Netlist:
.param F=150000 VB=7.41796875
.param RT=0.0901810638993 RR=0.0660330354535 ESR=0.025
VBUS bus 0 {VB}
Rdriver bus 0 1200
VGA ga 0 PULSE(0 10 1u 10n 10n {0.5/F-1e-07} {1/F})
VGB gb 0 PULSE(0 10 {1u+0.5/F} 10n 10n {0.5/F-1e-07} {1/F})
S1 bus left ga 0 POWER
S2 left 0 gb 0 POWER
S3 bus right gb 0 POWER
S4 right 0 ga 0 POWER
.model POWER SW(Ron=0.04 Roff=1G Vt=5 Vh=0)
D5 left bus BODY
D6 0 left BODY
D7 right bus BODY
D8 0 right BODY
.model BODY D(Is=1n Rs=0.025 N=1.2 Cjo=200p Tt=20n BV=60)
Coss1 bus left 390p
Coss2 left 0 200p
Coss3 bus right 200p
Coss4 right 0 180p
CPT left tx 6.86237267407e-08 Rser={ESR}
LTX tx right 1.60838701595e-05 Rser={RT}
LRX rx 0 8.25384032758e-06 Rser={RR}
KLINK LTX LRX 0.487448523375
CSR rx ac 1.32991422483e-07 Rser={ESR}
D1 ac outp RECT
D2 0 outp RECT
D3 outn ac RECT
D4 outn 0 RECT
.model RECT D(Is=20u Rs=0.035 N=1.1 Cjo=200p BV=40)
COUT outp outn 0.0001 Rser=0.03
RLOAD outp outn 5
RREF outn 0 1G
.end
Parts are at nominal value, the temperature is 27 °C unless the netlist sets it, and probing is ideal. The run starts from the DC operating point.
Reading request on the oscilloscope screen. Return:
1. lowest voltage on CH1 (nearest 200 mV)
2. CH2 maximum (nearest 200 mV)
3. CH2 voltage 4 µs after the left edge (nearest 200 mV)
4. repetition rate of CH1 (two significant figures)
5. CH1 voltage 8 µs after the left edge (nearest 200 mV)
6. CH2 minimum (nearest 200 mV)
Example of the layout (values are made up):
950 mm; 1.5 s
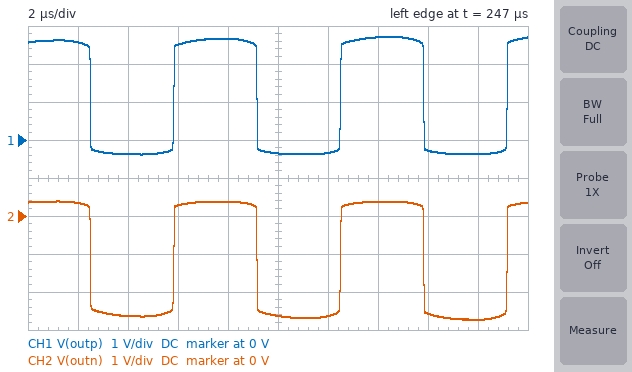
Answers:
-400 mV; 400 mV; -2.6 V; 150 kHz; 2.6 V; -2.8 V
